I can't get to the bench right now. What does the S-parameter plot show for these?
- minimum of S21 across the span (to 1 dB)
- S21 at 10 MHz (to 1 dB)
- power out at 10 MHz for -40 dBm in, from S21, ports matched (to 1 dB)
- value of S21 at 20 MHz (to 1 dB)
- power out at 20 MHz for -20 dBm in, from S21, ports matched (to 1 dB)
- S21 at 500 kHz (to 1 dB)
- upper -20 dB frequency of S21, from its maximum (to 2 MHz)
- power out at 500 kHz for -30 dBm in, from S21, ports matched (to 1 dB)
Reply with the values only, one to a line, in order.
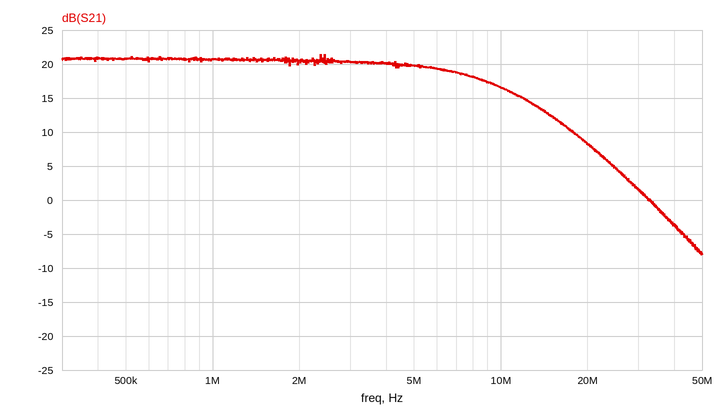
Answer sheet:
-8 dB
17 dB
-23 dBm
8 dB
-12 dBm
21 dB
30 MHz
-9 dBm
